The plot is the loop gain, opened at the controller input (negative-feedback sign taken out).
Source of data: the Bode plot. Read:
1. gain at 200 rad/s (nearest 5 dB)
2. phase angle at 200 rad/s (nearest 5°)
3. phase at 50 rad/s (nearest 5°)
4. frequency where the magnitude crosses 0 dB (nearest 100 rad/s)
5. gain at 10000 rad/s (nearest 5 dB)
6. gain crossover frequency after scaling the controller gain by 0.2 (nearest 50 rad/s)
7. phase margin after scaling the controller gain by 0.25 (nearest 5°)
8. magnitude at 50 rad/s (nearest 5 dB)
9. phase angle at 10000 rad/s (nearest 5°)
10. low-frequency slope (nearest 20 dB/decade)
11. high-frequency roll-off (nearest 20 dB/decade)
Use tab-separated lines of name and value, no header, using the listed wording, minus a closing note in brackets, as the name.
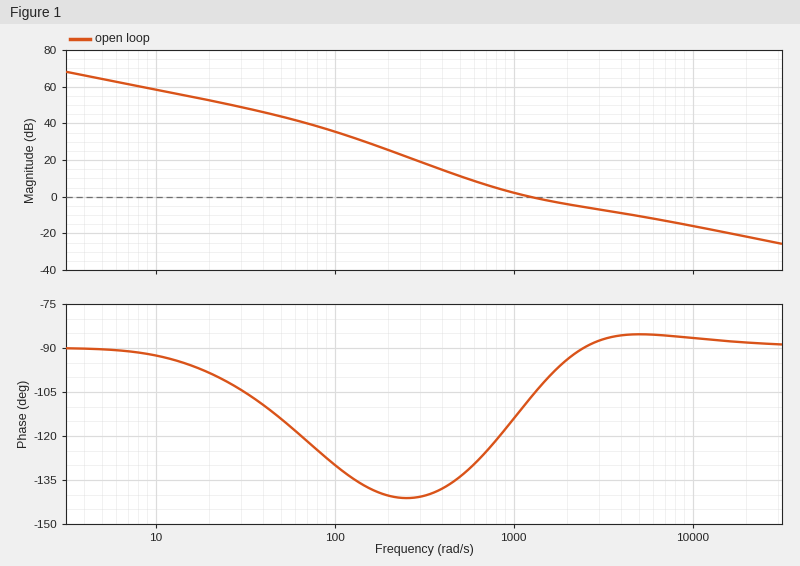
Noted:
gain at 200 rad/s	25 dB
phase angle at 200 rad/s	-140°
phase at 50 rad/s	-115°
frequency where the magnitude crosses 0 dB	1200 rad/s
gain at 10000 rad/s	-15 dB
gain crossover frequency after scaling the controller gain by 0.2	400 rad/s
phase margin after scaling the controller gain by 0.25	45°
magnitude at 50 rad/s	45 dB
phase angle at 10000 rad/s	-85°
low-frequency slope	-20 dB/decade
high-frequency roll-off	-20 dB/decade
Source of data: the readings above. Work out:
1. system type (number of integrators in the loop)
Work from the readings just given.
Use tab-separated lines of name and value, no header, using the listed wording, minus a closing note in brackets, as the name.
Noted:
system type	1
